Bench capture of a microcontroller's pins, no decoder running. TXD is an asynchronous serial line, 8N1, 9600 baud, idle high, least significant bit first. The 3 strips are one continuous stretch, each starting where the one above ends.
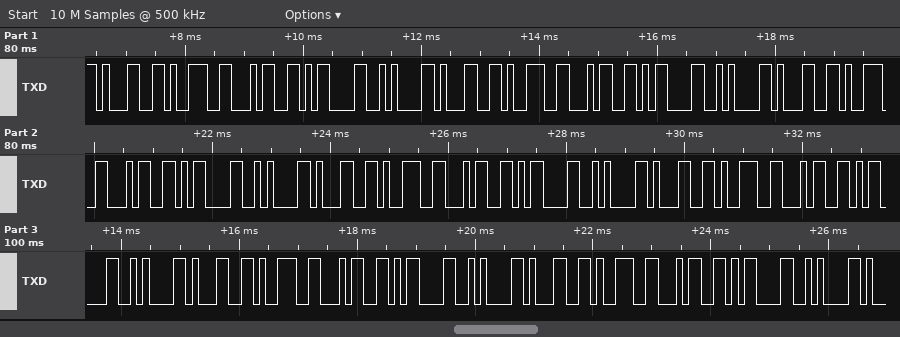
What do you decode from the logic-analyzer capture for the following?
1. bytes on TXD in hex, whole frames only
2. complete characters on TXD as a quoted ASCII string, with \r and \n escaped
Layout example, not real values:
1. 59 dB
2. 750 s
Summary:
1. 0x31 0x39 0x34 0x0D 0x0A 0x31 0x39 0x34 0x0D 0x0A 0x31 0x39 0x34 0x0D 0x0A 0x31 0x39 0x34 0x0D 0x0A 0x31 0x39 0x34 0x0D 0x0A 0x31 0x39 0x34 0x0D 0x0A 0x31 0x39 0x34 0x0D 0x0A
2. "194\r\n194\r\n194\r\n194\r\n194\r\n194\r\n194\r\n"
